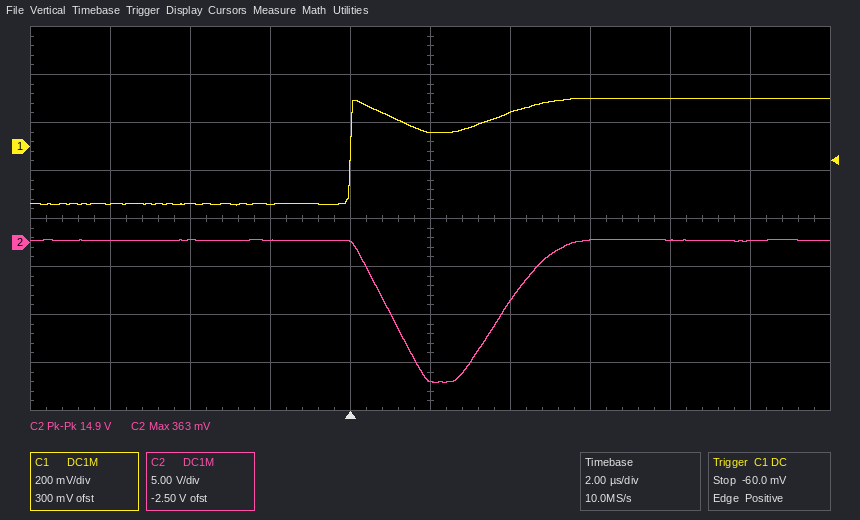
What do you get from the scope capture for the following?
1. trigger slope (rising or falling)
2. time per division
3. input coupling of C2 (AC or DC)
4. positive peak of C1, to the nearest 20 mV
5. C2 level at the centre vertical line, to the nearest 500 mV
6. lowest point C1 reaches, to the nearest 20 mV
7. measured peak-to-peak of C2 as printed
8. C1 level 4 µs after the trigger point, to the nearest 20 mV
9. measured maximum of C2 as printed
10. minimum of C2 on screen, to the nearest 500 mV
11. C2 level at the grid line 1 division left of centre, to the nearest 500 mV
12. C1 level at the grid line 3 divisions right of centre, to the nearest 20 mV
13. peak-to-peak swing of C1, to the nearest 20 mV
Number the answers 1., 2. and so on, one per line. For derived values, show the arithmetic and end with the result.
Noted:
1. rising
2. 2 µs
3. DC
4. 200 mV
5. -14.5 V
6. -240 mV
7. 14.9 V
8. 140 mV
9. 363 mV
10. -14.5 V
11. 0.0 V
12. 200 mV
13. 200 mV − (-240 mV) = 440 mV
